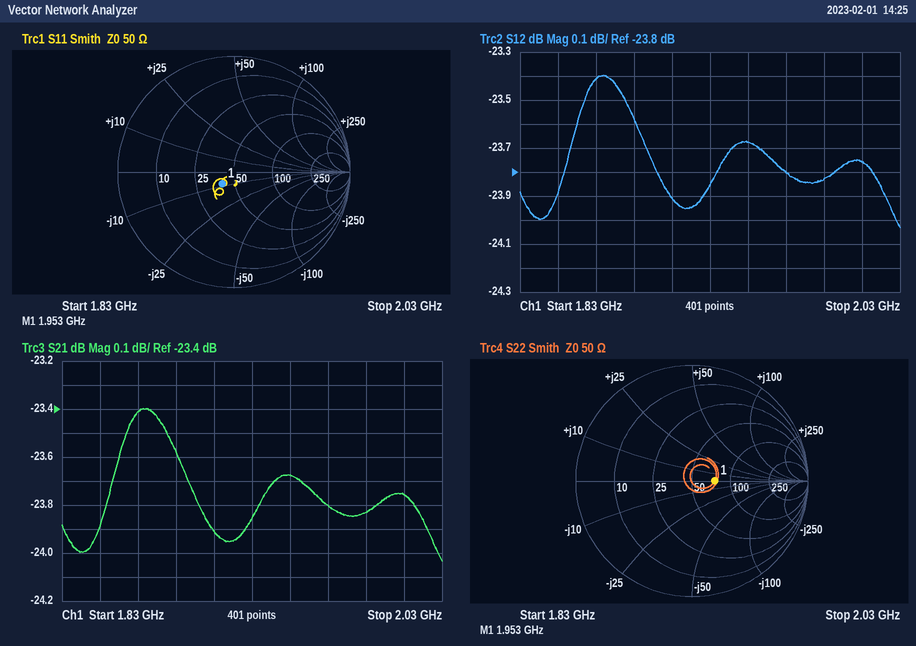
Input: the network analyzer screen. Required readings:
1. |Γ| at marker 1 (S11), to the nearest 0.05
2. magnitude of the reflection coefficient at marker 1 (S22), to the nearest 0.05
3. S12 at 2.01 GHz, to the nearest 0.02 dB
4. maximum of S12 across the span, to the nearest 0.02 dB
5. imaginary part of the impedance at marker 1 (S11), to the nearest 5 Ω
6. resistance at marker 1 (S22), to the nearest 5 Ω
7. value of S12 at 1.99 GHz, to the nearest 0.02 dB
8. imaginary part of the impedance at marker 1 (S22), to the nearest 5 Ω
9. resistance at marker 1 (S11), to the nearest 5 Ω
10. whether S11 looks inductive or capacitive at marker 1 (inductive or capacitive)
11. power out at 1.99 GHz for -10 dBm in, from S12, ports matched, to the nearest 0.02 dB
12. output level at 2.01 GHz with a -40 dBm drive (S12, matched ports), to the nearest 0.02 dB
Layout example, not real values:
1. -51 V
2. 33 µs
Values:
1. 0.15
2. 0.20
3. -23.76 dB
4. -23.40 dB
5. -10 Ω
6. 75 Ω
7. -23.82 dB
8. 0 Ω
9. 40 Ω
10. capacitive
11. -33.82 dBm
12. -63.76 dBm
